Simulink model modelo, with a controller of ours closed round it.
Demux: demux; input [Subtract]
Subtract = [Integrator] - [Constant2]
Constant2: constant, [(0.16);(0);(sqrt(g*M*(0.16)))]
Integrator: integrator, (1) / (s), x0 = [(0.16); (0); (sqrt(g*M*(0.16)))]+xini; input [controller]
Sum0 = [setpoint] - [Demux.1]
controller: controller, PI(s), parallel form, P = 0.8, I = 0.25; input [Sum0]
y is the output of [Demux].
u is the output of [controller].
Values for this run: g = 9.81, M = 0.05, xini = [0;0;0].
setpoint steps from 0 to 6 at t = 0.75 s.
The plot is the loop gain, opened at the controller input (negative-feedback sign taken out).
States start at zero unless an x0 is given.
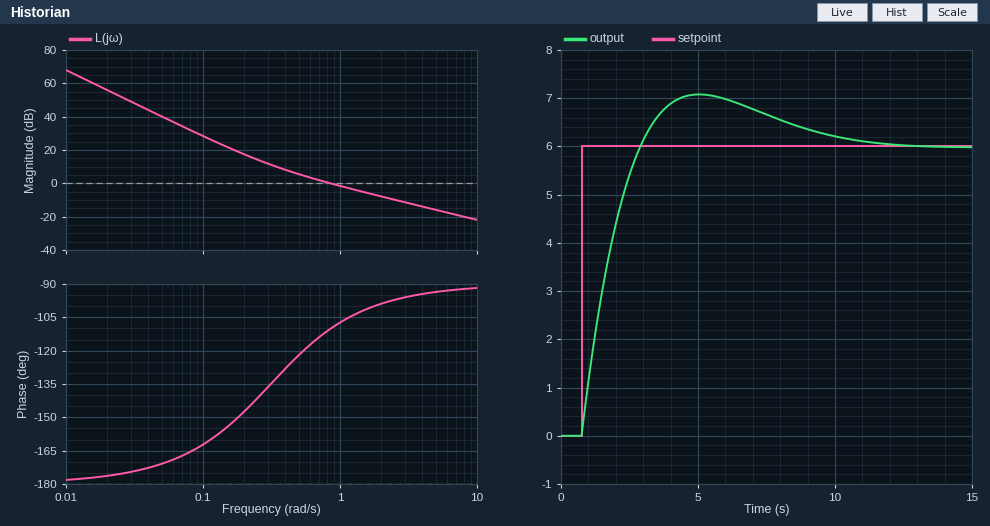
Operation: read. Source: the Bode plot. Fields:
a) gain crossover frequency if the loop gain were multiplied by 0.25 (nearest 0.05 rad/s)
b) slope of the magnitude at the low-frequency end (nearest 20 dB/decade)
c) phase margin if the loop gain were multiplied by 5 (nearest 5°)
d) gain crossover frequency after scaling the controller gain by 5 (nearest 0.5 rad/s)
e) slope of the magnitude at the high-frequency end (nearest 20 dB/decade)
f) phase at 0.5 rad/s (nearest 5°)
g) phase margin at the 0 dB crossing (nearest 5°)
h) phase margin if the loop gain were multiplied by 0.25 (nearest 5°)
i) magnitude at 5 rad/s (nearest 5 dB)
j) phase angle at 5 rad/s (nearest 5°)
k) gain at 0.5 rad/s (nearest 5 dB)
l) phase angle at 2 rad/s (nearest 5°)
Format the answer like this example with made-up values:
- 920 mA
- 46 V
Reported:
- 0.30 rad/s
- -40 dB/decade
- 85°
- 4.0 rad/s
- -20 dB/decade
- -120°
- 70°
- 45°
- -15 dB
- -95°
- 5 dB
- -100°
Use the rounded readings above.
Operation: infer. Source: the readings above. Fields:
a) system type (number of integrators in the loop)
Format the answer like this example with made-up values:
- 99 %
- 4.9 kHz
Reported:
- 2
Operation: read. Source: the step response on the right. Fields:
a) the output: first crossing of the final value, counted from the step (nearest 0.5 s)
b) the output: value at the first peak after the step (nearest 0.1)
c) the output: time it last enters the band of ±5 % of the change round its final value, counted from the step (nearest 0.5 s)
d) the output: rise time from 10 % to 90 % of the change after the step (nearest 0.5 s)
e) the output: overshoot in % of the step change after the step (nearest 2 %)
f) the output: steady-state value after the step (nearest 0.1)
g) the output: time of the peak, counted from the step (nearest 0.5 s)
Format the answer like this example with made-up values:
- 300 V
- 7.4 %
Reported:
- 2.0 s
- 7.1
- 8.5 s
- 1.5 s
- 18 %
- 6.0
- 4.5 s
